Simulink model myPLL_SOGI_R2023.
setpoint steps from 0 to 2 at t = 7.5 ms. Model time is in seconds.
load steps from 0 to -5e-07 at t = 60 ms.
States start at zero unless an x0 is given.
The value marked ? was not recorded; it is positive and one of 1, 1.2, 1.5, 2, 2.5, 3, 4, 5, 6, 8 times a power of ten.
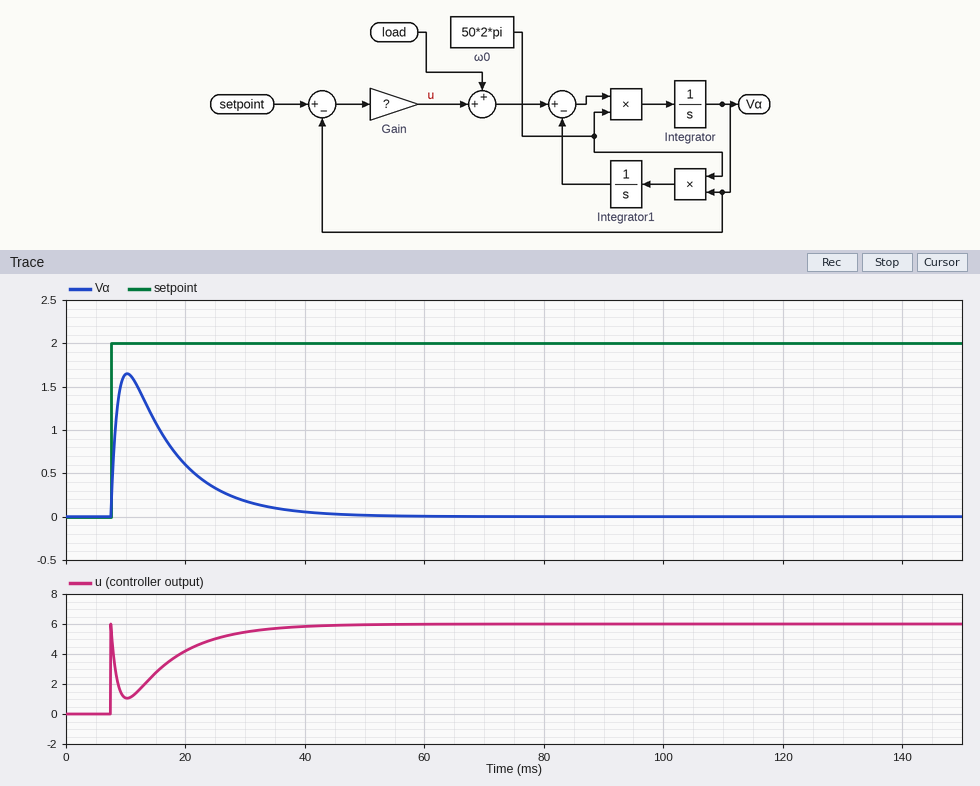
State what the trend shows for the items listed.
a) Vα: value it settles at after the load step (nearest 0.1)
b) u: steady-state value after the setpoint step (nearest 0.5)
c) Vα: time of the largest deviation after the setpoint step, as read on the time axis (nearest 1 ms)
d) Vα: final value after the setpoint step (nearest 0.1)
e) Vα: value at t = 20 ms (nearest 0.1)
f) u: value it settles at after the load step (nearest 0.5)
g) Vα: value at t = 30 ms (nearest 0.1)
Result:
0.0
6.0
10 ms
0.0
0.6
6.0
0.2
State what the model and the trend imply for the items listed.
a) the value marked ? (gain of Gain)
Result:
3
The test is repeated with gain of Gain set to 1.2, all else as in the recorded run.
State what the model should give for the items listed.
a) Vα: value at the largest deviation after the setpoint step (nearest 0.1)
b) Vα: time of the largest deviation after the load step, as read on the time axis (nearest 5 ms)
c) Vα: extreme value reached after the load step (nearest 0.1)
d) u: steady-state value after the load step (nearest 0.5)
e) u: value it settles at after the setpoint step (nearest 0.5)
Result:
1.2
75 ms
0.0
2.5
2.5
